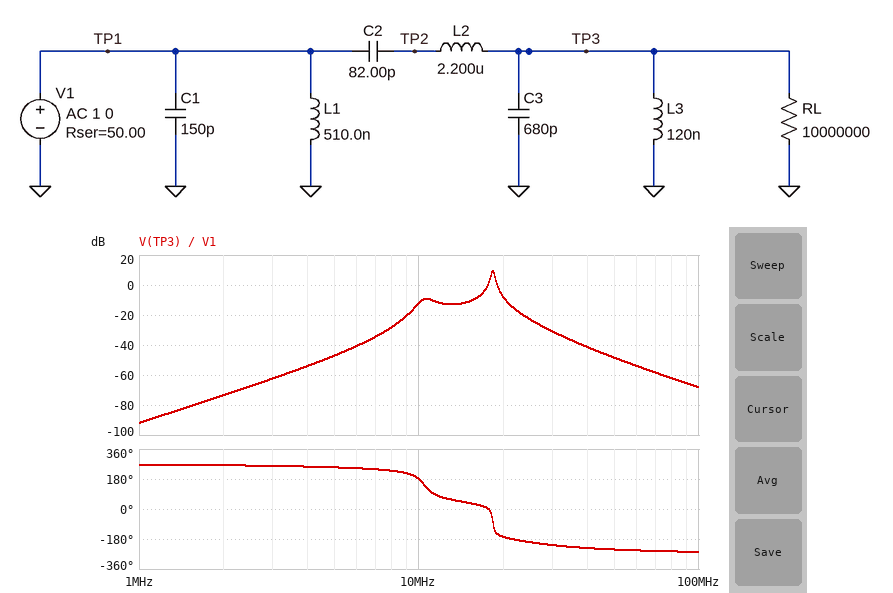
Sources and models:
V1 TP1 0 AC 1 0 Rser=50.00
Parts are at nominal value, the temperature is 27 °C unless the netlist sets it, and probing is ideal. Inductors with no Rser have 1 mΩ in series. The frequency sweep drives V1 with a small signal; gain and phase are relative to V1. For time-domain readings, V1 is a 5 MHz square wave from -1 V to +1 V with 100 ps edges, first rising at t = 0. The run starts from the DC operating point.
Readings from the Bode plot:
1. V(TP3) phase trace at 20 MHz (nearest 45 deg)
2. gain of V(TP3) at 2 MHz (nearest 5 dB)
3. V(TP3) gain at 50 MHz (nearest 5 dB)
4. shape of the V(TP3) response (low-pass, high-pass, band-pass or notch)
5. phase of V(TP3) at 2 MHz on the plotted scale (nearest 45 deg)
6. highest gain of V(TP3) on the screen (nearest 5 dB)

-180 deg
-75 dB
-50 dB
band-pass
270 deg
10 dB
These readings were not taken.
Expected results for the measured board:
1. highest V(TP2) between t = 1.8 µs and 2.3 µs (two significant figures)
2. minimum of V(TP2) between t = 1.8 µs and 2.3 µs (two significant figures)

1.1 V
-1.1 V
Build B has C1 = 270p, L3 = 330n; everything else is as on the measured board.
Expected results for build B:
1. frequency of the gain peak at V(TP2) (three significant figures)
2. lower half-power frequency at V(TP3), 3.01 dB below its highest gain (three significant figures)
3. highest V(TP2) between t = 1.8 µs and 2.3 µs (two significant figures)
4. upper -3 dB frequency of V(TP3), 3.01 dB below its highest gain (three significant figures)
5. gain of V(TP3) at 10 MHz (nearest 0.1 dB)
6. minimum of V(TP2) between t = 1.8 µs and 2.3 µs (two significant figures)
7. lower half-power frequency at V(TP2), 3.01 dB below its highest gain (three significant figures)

9.02 MHz
8.77 MHz
1.4 V
9.48 MHz
-0.3 dB
-1.4 V
8.72 MHz
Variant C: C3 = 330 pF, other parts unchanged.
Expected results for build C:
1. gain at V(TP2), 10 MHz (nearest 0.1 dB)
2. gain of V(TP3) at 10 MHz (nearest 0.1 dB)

9.9 dB
-14.4 dB
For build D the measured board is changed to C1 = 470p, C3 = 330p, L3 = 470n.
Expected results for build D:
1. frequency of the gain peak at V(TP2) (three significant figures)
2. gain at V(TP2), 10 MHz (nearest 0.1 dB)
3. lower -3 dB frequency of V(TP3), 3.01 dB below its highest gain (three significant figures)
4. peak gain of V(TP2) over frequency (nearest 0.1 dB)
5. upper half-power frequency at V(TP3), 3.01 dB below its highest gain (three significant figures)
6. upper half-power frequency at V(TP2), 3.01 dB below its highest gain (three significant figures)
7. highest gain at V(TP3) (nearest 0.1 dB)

16.2 MHz
11.7 dB
15.7 MHz
14.0 dB
16.5 MHz
16.6 MHz
8.9 dB
